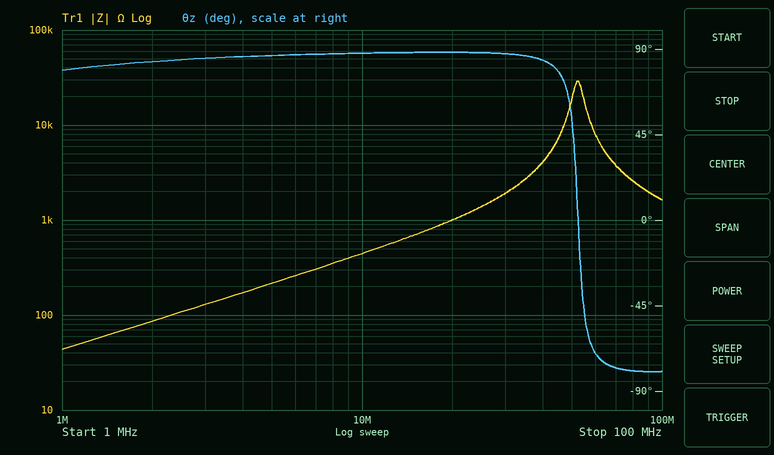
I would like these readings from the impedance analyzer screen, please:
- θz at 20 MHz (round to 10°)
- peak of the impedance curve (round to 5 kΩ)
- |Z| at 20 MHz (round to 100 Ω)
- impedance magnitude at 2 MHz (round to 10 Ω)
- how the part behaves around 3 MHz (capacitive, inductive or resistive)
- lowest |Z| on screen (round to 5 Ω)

90°
30 kΩ
1.0 kΩ
90 Ω
inductive
45 Ω
